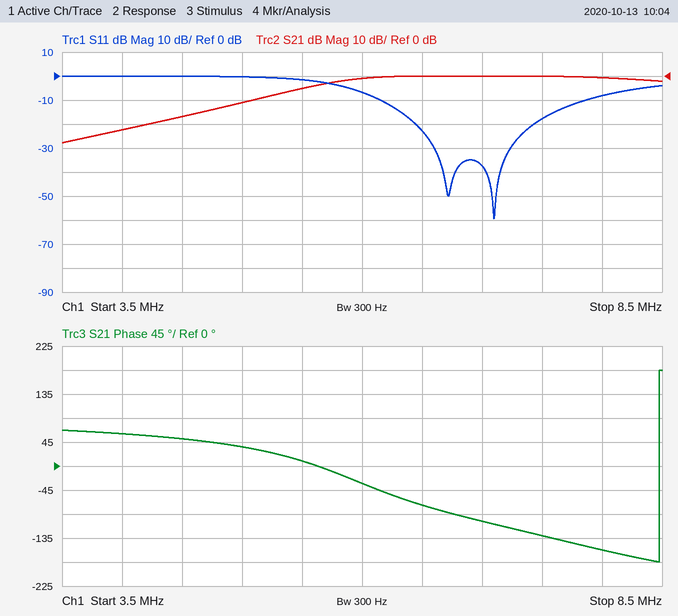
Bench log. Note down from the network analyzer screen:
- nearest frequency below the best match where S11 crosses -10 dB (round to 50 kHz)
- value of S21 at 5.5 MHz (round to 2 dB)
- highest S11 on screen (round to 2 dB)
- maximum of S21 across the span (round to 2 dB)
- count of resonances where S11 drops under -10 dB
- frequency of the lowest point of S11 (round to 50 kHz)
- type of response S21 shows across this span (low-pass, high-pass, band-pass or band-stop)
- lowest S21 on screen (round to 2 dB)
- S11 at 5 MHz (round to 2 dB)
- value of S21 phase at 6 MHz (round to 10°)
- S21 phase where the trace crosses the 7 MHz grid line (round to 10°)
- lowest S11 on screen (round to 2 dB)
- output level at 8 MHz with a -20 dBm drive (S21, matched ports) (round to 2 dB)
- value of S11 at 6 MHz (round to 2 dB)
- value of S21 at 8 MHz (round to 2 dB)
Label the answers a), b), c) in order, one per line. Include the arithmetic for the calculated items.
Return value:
a) 6.15 MHz
b) -6 dB
c) 0 dB
d) 0 dB
e) 2
f) 7.10 MHz
g) high-pass
h) -28 dB
i) 0 dB
j) -30°
k) -100°
l) -60 dB
m) -20 dBm + (0 dB) = -20 dBm
n) -6 dB
o) 0 dB
